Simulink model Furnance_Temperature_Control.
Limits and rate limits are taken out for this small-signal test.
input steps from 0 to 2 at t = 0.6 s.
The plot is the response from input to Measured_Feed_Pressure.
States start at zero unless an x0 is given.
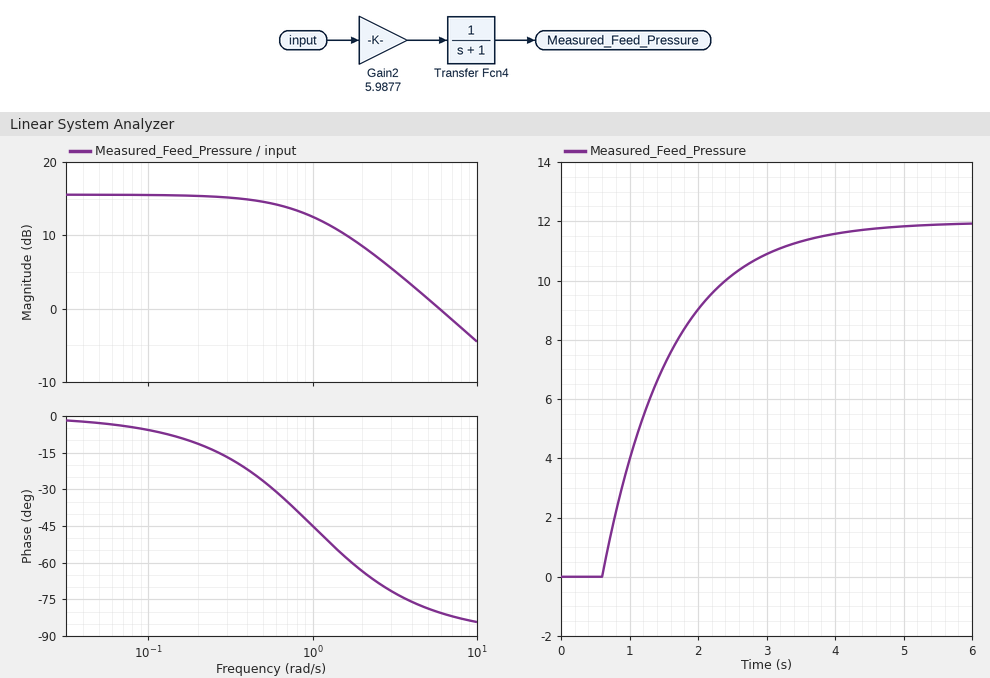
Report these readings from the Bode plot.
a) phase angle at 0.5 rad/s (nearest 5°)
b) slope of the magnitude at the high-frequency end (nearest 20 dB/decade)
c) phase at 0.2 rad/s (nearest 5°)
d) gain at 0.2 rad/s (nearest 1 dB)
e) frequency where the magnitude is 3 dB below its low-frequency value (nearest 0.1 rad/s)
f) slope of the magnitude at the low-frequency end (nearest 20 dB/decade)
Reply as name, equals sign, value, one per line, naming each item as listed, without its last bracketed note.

phase angle at 0.5 rad/s = -25°
slope of the magnitude at the high-frequency end = -20 dB/decade
phase at 0.2 rad/s = -10°
gain at 0.2 rad/s = 15 dB
frequency where the magnitude is 3 dB below its low-frequency value = 1.0 rad/s
slope of the magnitude at the low-frequency end = 0 dB/decade
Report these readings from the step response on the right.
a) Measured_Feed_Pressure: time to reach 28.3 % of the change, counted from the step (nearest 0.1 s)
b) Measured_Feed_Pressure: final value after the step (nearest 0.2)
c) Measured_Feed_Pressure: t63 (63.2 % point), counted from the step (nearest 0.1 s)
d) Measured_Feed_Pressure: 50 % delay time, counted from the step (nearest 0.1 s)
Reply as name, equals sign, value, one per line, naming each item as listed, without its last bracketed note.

Measured_Feed_Pressure: time to reach 28.3 % of the change, counted from the step = 0.3 s
Measured_Feed_Pressure: final value after the step = 12.0
Measured_Feed_Pressure: t63 (63.2 % point), counted from the step = 1.0 s
Measured_Feed_Pressure: 50 % delay time, counted from the step = 0.7 s
